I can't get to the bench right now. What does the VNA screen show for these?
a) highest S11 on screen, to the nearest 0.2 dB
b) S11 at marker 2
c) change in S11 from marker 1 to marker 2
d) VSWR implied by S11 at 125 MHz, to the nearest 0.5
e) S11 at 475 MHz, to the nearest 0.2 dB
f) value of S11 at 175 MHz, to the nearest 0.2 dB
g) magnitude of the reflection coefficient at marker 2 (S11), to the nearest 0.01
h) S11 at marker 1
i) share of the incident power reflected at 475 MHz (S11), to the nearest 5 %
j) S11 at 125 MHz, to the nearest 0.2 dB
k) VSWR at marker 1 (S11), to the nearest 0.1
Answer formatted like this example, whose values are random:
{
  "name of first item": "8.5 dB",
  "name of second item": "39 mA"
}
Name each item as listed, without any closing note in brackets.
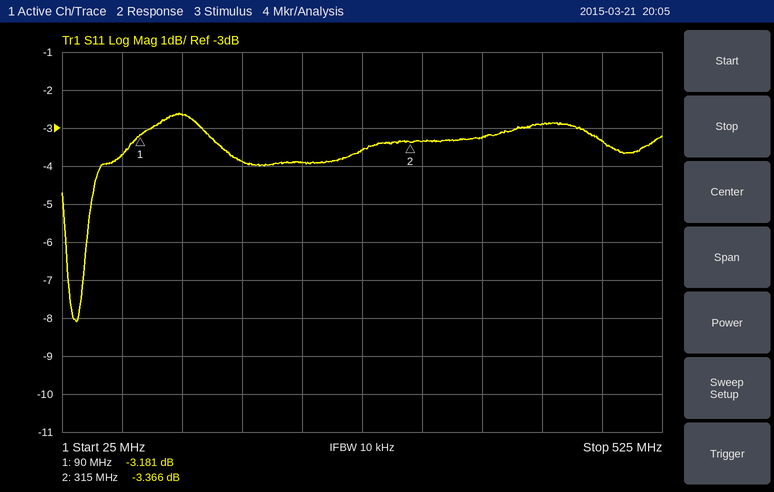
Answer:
{
  "highest S11 on screen, to the nearest 0.2 dB": "-2.6 dB",
  "S11 at marker 2": "-3.366 dB",
  "change in S11 from marker 1 to marker 2": "-0.185 dB",
  "VSWR implied by S11 at 125 MHz, to the nearest 0.5": "6.5",
  "S11 at 475 MHz, to the nearest 0.2 dB": "-3.4 dB",
  "value of S11 at 175 MHz, to the nearest 0.2 dB": "-3.8 dB",
  "magnitude of the reflection coefficient at marker 2 (S11), to the nearest 0.01": "0.68",
  "S11 at marker 1": "-3.181 dB",
  "share of the incident power reflected at 475 MHz (S11), to the nearest 5 %": "45 %",
  "S11 at 125 MHz, to the nearest 0.2 dB": "-2.6 dB",
  "VSWR at marker 1 (S11), to the nearest 0.1": "5.5"
}
